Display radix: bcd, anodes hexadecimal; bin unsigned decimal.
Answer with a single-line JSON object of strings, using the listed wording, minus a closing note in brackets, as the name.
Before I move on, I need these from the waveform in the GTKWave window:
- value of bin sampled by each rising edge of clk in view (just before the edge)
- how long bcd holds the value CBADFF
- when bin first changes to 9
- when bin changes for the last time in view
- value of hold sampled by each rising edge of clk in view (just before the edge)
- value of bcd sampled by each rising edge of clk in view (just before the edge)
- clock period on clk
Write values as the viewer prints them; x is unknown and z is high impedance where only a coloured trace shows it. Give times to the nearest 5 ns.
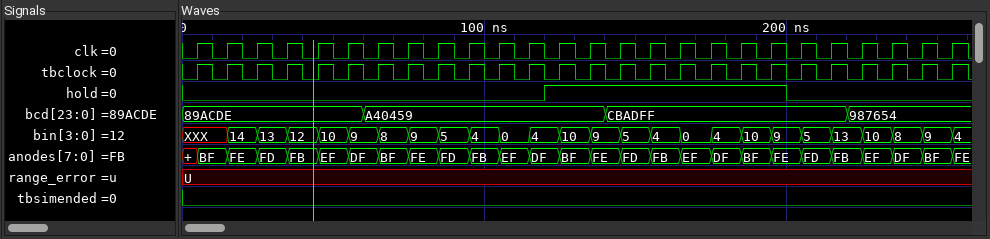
{"value of bin sampled by each rising edge of clk in view": "XXX, XXX, 14, 13, 12, 10, 9, 8, 9, 5, 4, 0, 4, 10, 9, 5, 4, 0, 4, 10, 9, 5, 13, 10, 8, 9", "how long bcd holds the value CBADFF": "80 ns", "when bin first changes to 9": "55 ns", "when bin changes for the last time in view": "255 ns", "value of hold sampled by each rising edge of clk in view": "0 0 0 0 0 0 0 0 0 0 0 0 1 1 1 1 1 1 1 1 0 0 0 0 0 0", "value of bcd sampled by each rising edge of clk in view": "89ACDE, 89ACDE, 89ACDE, 89ACDE, 89ACDE, 89ACDE, A40459, A40459, A40459, A40459, A40459, A40459, A40459, A40459, CBADFF, CBADFF, CBADFF, CBADFF, CBADFF, CBADFF, CBADFF, CBADFF, 987654, 987654, 987654, 987654", "clock period on clk": "10 ns"}
